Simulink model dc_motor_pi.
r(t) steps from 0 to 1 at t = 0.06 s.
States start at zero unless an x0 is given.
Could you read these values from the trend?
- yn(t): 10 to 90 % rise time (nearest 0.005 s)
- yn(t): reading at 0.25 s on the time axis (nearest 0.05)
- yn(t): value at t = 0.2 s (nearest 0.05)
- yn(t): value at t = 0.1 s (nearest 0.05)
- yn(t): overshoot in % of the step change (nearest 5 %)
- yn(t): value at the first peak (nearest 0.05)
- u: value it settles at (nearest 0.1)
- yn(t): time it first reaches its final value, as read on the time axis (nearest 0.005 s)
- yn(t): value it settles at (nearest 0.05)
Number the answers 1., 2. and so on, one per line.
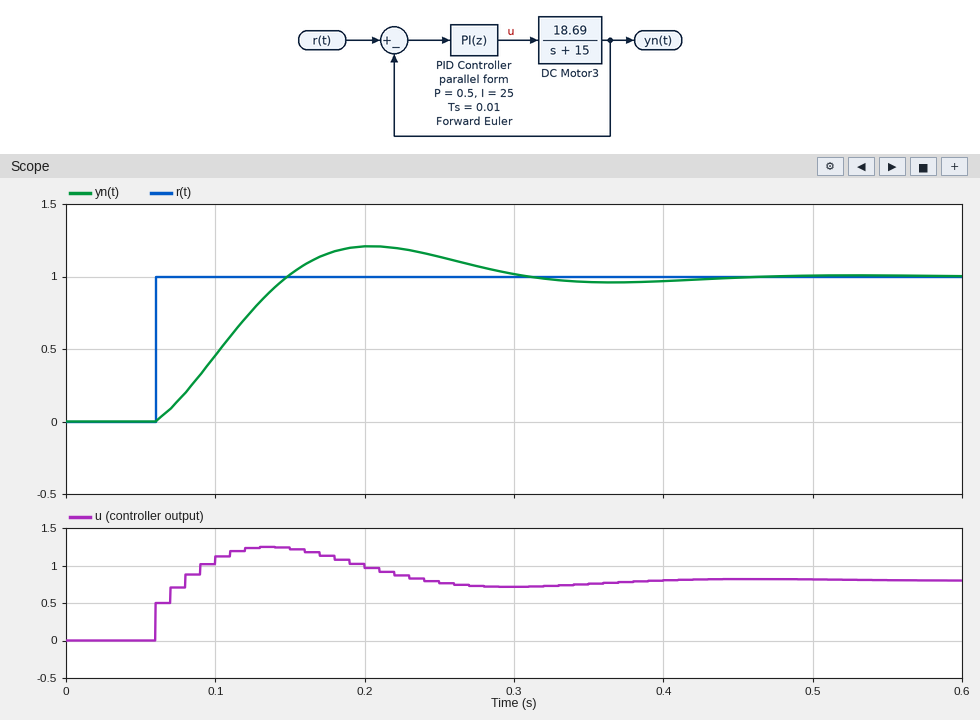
1. 0.065 s
2. 1.15
3. 1.20
4. 0.45
5. 20 %
6. 1.20
7. 0.8
8. 0.150 s
9. 1.00
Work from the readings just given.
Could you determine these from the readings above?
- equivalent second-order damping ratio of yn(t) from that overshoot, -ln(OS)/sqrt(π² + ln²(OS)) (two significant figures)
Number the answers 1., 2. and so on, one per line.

1. 0.46
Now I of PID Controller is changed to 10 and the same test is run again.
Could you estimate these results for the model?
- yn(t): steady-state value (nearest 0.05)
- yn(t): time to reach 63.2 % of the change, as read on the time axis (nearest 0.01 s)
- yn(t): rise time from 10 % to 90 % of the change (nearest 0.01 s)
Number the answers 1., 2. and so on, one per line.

1. 1.00
2. 0.15 s
3. 0.15 s
